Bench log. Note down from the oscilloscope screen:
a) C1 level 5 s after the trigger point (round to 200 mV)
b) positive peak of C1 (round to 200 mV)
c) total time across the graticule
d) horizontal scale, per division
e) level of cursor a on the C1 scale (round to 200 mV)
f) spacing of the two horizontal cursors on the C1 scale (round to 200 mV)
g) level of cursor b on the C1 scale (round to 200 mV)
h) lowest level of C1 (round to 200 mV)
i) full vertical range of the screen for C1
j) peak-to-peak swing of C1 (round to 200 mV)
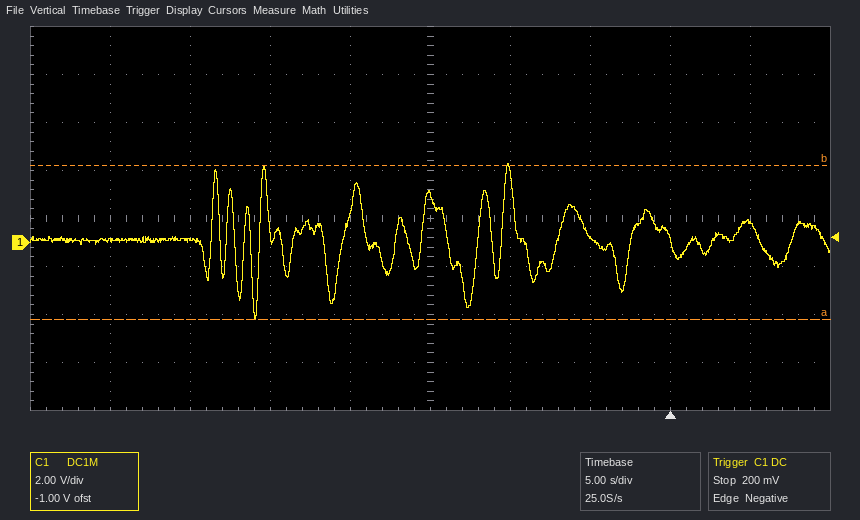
800 mV
3.2 V
50 s
5 s
-3.2 V
6.4 V
3.2 V
-3.2 V
16 V
6.4 V
